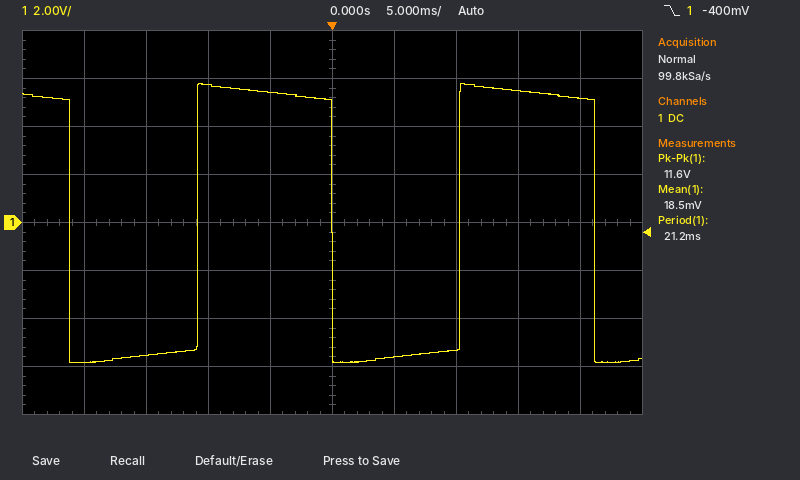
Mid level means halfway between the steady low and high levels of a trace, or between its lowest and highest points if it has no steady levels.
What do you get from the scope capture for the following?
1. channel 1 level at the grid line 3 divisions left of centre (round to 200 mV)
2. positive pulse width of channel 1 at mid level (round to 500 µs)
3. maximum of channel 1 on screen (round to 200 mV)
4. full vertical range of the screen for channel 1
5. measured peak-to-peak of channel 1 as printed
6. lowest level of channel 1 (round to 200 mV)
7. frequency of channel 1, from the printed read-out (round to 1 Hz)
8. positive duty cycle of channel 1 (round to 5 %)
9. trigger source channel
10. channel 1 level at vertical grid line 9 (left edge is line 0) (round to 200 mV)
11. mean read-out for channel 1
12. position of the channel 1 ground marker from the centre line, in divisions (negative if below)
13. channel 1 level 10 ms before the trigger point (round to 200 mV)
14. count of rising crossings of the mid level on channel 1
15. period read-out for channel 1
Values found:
-5.6 V
11.0 ms
5.8 V
16 V
11.6 V
-5.8 V
47 Hz
50 %
channel 1
5.2 V
18.5 mV
0.0 div
5.8 V
2
21.2 ms
